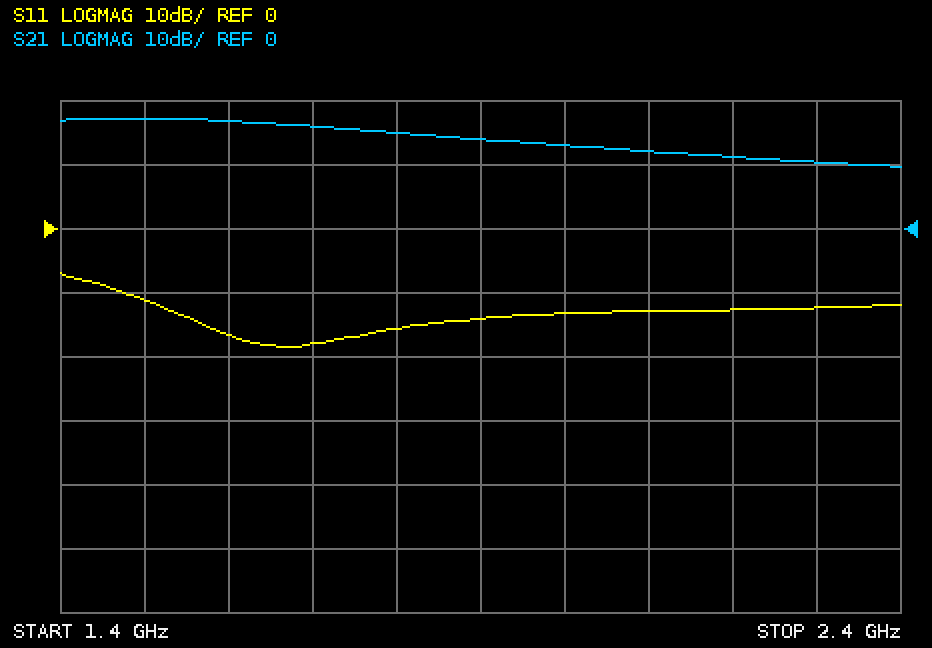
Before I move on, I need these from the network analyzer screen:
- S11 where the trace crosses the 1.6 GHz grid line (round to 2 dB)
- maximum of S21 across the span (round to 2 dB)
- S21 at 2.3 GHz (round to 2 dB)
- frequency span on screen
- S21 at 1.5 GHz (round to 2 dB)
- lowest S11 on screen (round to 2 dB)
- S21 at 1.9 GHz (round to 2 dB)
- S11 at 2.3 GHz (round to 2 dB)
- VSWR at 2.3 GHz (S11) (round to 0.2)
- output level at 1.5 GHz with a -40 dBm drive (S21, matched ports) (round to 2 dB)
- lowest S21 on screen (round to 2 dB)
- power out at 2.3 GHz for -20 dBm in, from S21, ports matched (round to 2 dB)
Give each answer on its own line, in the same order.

-16 dB
18 dB
10 dB
1 GHz
18 dB
-18 dB
14 dB
-12 dB
1.6
-22 dBm
10 dB
-10 dBm
